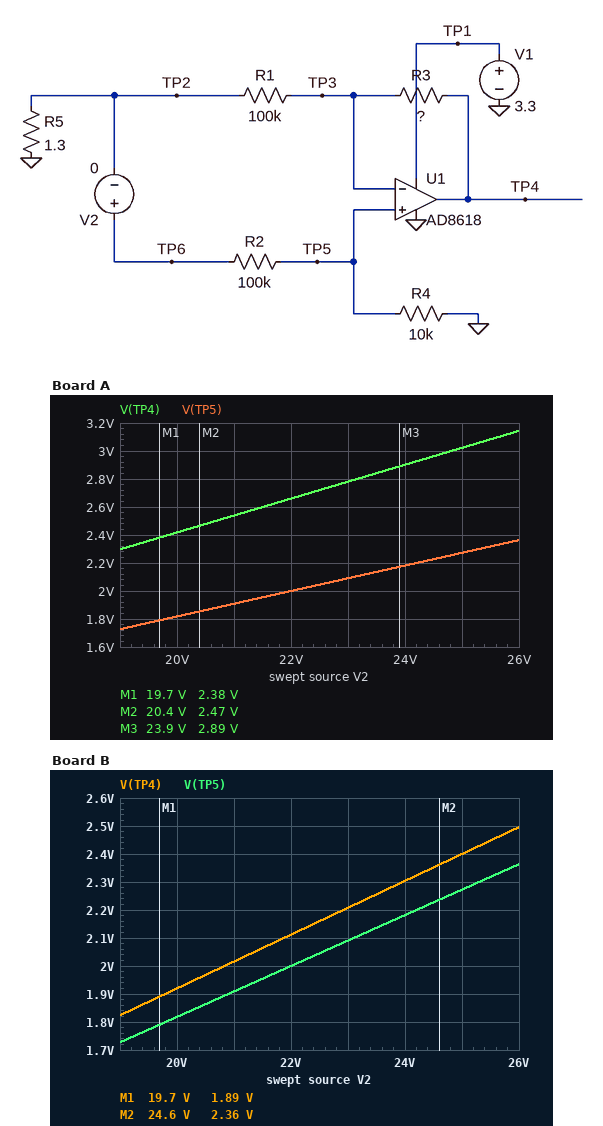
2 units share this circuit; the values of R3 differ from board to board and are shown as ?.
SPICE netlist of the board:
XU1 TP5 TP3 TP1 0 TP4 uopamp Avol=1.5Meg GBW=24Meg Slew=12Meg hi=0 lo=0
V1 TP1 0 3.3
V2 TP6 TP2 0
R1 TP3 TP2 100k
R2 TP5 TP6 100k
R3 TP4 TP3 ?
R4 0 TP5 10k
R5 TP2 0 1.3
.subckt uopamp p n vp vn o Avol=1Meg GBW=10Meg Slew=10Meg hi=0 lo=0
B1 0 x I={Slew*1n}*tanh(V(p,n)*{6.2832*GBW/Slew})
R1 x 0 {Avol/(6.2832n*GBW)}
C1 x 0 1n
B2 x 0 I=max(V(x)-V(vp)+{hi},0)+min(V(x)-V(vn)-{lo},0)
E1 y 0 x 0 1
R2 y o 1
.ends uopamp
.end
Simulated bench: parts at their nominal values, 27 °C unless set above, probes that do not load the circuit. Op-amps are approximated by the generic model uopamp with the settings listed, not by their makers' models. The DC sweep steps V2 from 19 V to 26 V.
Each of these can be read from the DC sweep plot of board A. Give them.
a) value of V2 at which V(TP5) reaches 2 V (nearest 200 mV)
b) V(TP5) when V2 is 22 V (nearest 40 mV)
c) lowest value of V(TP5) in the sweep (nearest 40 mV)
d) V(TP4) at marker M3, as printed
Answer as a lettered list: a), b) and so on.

a) 22.0 V
b) 2.00 V
c) 1.72 V
d) 2.89 V
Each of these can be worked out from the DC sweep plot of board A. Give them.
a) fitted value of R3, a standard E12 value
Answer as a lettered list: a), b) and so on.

a) 33 kΩ
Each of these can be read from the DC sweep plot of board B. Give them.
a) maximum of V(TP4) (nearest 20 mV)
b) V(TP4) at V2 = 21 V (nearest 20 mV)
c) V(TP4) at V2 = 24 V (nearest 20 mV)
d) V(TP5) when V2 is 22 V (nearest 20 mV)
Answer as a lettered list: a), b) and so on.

a) 2.50 V
b) 2.02 V
c) 2.30 V
d) 2.00 V
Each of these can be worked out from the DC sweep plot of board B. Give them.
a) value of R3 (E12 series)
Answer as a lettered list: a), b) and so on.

a) 5.6 kΩ
